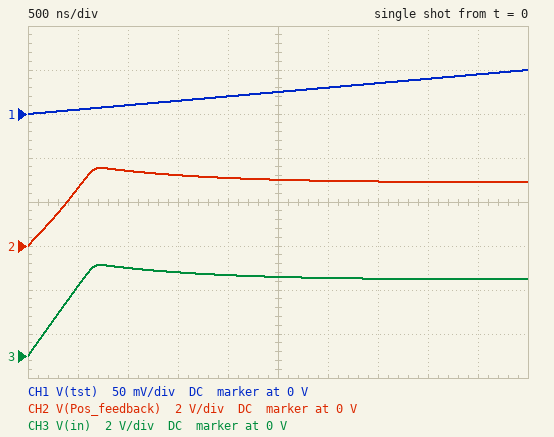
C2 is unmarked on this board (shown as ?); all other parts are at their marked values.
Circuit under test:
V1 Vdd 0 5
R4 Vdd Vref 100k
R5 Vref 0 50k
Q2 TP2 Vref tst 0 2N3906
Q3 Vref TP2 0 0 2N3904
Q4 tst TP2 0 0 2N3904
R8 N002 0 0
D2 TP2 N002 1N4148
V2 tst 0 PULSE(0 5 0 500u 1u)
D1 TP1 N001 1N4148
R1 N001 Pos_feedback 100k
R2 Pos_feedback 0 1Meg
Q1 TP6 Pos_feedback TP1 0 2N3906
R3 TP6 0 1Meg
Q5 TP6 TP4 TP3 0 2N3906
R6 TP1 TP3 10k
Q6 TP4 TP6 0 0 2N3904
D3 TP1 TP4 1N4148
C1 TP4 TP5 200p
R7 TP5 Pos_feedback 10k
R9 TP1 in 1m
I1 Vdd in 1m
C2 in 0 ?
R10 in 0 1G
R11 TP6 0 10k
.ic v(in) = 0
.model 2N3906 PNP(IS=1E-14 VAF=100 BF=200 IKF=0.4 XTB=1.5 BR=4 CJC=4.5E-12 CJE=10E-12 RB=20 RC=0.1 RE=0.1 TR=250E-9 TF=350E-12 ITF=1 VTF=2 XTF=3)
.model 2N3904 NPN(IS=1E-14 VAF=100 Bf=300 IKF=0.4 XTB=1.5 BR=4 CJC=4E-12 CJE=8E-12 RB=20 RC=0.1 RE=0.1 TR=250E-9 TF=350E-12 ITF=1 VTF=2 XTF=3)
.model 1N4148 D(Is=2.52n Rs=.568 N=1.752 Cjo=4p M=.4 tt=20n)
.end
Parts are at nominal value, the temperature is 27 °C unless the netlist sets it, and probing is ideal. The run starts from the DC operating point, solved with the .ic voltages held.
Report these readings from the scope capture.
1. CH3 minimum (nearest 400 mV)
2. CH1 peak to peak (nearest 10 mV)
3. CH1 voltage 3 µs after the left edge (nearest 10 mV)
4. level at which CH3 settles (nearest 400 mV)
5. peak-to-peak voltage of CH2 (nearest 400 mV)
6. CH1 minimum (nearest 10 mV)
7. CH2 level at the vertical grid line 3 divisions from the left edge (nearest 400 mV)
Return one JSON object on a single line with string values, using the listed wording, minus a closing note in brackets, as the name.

{"CH3 minimum": "0 V", "CH1 peak to peak": "50 mV", "CH1 voltage 3 µs after the left edge": "30 mV", "level at which CH3 settles": "3.6 V", "peak-to-peak voltage of CH2": "3.6 V", "CH1 minimum": "0 V", "CH2 level at the vertical grid line 3 divisions from the left edge": "3.2 V"}
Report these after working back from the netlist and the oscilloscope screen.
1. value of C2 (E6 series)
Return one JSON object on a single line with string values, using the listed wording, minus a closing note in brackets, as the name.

{"value of C2": "150 pF"}
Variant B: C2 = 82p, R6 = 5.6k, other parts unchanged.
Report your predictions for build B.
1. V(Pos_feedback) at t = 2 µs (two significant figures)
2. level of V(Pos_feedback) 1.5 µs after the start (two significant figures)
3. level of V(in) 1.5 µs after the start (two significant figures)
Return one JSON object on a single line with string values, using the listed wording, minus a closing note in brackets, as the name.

{"V(Pos_feedback) at t = 2 µs": "2.9 V", "level of V(Pos_feedback) 1.5 µs after the start": "2.8 V", "level of V(in) 1.5 µs after the start": "3.4 V"}
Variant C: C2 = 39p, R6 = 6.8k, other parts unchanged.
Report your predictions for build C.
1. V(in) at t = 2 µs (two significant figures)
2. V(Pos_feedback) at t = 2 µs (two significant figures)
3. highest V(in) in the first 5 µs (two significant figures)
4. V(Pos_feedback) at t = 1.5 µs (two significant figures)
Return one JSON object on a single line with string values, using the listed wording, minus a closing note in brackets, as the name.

{"V(in) at t = 2 µs": "3.4 V", "V(Pos_feedback) at t = 2 µs": "2.9 V", "highest V(in) in the first 5 µs": "3.6 V", "V(Pos_feedback) at t = 1.5 µs": "2.8 V"}
